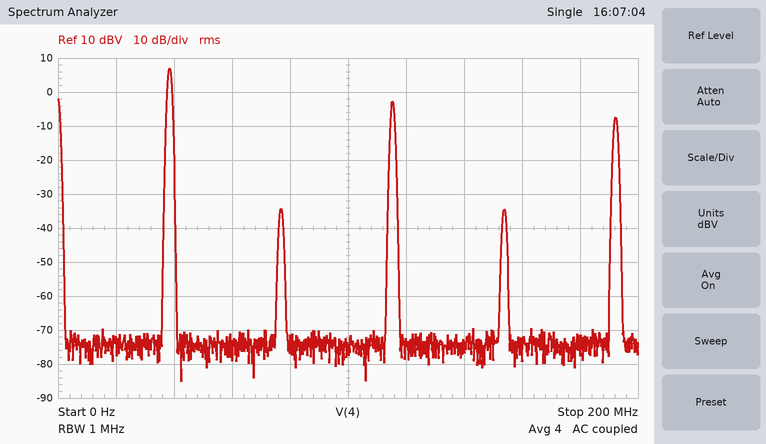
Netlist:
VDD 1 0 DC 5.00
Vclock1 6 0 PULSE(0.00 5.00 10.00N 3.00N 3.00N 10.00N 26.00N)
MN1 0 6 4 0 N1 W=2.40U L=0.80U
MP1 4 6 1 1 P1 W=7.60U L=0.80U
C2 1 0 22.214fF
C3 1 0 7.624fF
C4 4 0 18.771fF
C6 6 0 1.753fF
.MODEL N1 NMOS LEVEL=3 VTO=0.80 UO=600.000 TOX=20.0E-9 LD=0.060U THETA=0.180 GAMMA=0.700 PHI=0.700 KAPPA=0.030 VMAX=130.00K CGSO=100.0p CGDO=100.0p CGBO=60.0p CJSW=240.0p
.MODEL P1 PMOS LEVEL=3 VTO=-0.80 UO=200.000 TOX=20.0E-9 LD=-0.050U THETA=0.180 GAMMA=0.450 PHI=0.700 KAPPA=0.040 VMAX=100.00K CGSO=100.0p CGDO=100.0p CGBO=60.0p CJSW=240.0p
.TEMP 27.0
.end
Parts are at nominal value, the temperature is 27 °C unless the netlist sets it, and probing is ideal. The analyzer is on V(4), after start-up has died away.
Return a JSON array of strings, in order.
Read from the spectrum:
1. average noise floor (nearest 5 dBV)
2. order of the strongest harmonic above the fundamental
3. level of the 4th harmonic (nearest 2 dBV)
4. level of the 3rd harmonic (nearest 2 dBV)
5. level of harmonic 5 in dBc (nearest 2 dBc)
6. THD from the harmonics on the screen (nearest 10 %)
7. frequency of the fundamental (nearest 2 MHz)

["-75 dBV", "3", "-34 dBV", "-2 dBV", "-14 dBc", "40 %", "38 MHz"]
